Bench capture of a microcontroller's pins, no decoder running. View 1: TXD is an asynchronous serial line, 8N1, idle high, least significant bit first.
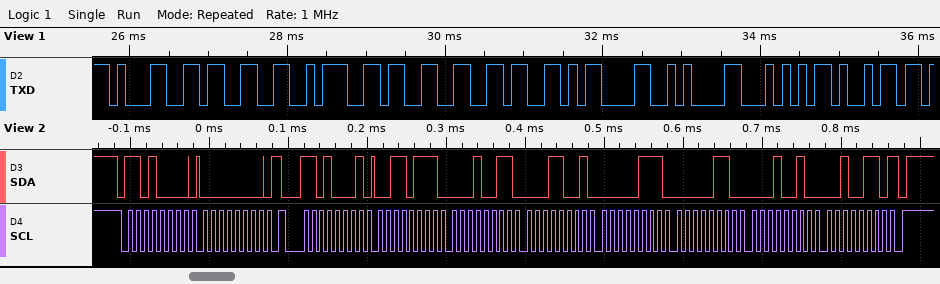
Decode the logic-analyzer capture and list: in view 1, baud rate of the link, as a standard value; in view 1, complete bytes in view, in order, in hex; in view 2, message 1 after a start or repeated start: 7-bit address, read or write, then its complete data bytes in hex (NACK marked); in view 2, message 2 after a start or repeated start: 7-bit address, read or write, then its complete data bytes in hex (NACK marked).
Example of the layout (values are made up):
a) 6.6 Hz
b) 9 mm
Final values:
a) 9600 baud
b) 31 33 3A 33 36 0D 0A 54 69
c) 0x68 write: 00
d) 0x68 read: 37 13 19 07 06 12 26 NACK
